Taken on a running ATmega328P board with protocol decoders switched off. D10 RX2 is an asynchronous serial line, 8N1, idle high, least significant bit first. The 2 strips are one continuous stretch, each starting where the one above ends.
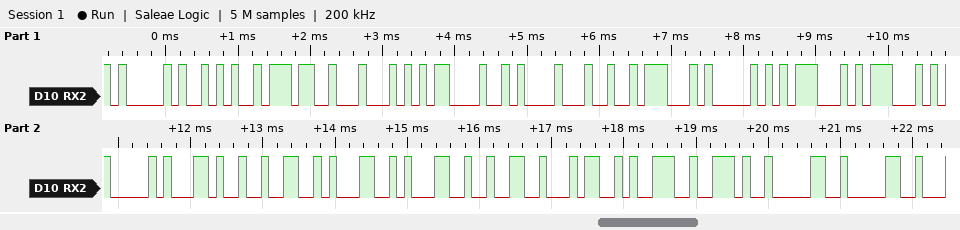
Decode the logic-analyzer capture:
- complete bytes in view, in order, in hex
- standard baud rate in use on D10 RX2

41 2A 37 44 0D 0A 24 47 50 47 47 41 2C 32 31 31 32 34 39 2E 30 30
9600 baud
